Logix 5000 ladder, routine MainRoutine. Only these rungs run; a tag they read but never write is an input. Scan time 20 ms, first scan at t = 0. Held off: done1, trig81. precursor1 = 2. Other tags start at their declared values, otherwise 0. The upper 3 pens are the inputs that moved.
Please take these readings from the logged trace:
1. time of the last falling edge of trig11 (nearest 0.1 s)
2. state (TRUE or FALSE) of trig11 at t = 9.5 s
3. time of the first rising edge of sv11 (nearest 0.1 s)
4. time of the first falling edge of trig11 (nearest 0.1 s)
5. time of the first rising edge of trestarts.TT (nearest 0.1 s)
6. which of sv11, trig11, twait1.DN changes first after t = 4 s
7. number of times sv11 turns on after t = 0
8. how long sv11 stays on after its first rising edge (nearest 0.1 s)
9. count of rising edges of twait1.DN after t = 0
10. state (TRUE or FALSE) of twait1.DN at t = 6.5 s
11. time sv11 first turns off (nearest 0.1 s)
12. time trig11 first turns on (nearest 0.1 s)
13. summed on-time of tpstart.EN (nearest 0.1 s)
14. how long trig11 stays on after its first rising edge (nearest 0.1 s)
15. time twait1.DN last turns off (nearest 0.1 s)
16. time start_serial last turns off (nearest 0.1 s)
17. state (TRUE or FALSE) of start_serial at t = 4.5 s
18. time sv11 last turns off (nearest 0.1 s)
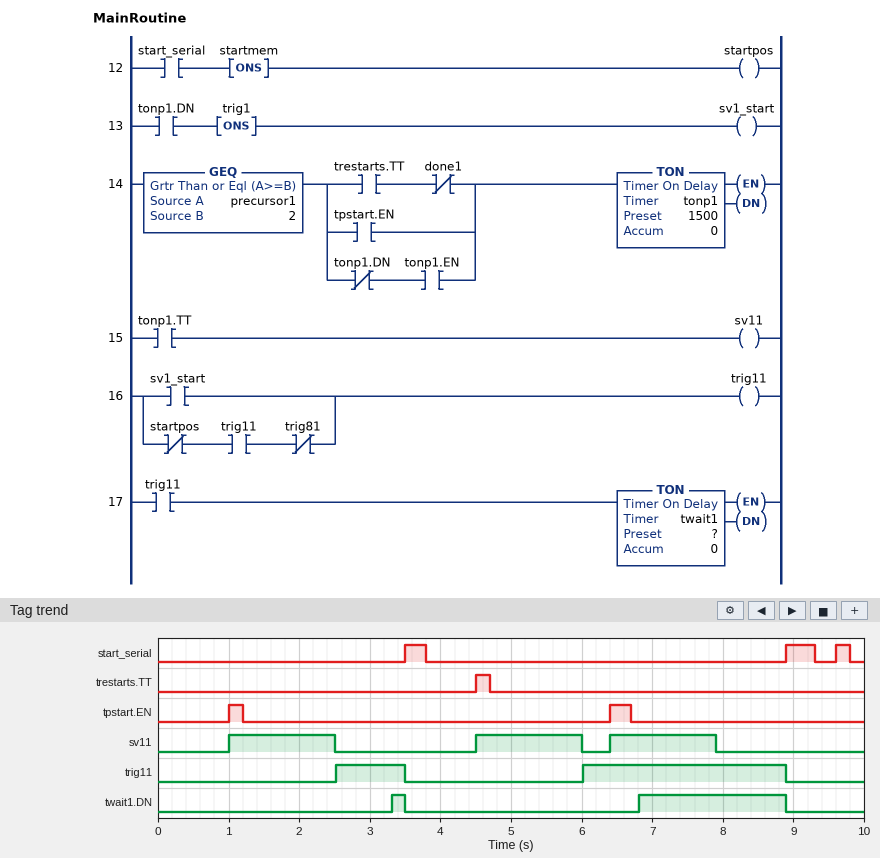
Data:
8.9 s
FALSE
1.0 s
3.5 s
4.5 s
sv11
3
1.5 s
2
FALSE
2.5 s
2.5 s
0.5 s
1.0 s
8.9 s
9.8 s
FALSE
7.9 s
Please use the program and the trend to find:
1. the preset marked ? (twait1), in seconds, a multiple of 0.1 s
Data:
0.8 s
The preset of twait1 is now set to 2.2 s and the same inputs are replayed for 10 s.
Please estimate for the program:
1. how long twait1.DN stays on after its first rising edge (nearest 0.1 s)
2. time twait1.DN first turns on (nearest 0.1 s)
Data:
0.7 s
8.2 s
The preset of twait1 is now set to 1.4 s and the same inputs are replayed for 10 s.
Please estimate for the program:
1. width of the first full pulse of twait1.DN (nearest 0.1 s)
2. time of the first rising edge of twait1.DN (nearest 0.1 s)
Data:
1.5 s
7.4 s
